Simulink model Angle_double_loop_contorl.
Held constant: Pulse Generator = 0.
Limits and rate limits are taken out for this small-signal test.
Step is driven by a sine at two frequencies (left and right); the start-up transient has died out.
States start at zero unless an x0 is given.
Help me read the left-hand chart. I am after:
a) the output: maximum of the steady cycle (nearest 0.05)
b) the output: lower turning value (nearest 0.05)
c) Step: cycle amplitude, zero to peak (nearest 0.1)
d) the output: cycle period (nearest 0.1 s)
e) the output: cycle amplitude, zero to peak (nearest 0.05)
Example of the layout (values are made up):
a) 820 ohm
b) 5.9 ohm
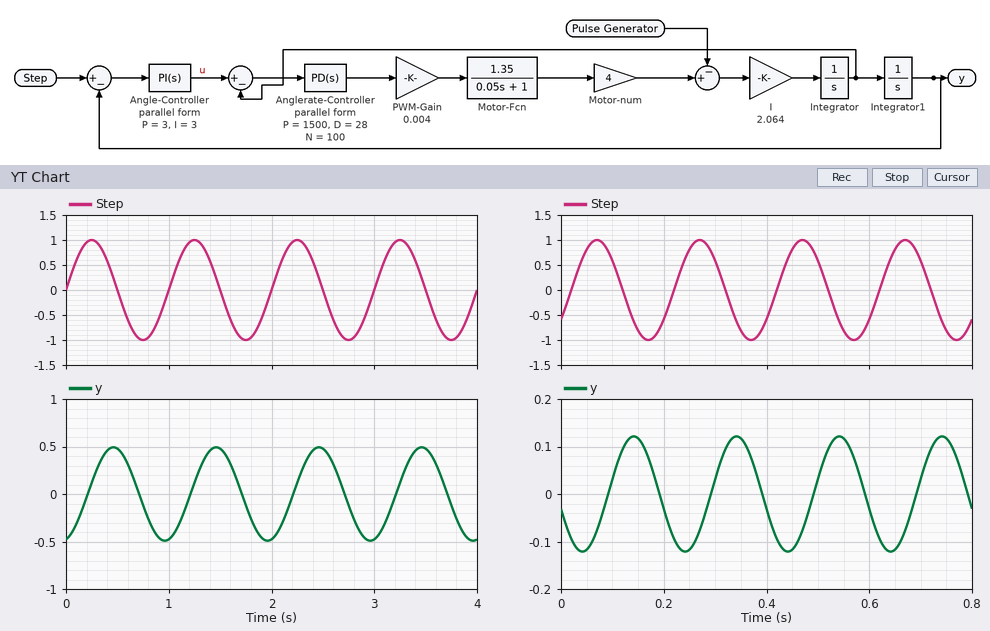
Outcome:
a) 0.50
b) -0.50
c) 1.0
d) 1.0 s
e) 0.50
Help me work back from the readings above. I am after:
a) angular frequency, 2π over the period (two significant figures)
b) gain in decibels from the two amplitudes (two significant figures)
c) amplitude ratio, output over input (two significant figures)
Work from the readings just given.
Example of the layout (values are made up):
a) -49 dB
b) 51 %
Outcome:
a) 6.3 rad/s
b) -6.0 dB
c) 0.50
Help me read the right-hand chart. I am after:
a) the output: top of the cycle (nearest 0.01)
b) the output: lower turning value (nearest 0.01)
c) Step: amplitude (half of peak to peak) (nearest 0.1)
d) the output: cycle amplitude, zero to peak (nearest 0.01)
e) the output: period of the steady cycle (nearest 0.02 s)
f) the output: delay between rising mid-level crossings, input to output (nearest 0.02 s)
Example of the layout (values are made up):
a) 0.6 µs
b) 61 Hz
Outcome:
a) 0.12
b) -0.12
c) 1.0
d) 0.12
e) 0.20 s
f) 0.08 s
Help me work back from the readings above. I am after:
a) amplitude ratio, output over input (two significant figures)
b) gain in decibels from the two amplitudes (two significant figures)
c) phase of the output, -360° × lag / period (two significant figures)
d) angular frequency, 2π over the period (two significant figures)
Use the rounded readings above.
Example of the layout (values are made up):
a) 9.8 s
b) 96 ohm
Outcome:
a) 0.12
b) -18 dB
c) -140°
d) 31 rad/s
